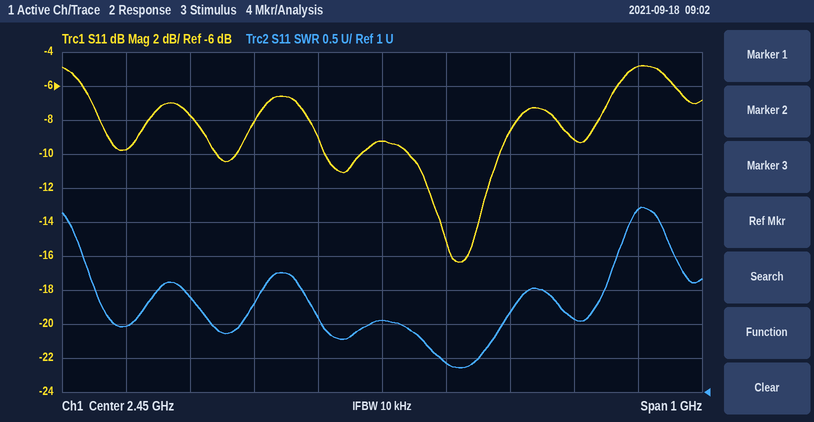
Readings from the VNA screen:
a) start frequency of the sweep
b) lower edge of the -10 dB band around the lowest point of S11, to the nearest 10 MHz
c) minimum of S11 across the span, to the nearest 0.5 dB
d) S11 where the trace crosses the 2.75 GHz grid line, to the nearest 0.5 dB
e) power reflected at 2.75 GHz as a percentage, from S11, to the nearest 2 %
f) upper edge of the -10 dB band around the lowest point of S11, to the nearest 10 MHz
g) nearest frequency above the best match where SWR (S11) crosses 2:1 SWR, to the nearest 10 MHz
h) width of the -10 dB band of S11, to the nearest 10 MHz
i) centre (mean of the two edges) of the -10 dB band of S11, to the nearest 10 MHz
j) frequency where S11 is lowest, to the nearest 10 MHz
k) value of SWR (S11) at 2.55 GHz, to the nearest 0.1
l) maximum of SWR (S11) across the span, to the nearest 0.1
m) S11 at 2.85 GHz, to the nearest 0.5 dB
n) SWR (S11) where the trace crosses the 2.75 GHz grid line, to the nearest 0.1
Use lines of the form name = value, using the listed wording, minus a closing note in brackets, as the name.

start frequency of the sweep = 1.95 GHz
lower edge of the -10 dB band around the lowest point of S11, to the nearest 10 MHz = 2.49 GHz
minimum of S11 across the span, to the nearest 0.5 dB = -16.5 dB
S11 where the trace crosses the 2.75 GHz grid line, to the nearest 0.5 dB = -9.0 dB
power reflected at 2.75 GHz as a percentage, from S11, to the nearest 2 % = 12 %
upper edge of the -10 dB band around the lowest point of S11, to the nearest 10 MHz = 2.63 GHz
nearest frequency above the best match where SWR (S11) crosses 2:1 SWR, to the nearest 10 MHz = 2.64 GHz
width of the -10 dB band of S11, to the nearest 10 MHz = 140 MHz
centre (mean of the two edges) of the -10 dB band of S11, to the nearest 10 MHz = 2.56 GHz
frequency where S11 is lowest, to the nearest 10 MHz = 2.57 GHz
value of SWR (S11) at 2.55 GHz, to the nearest 0.1 = 1.4
maximum of SWR (S11) across the span, to the nearest 0.1 = 3.7
S11 at 2.85 GHz, to the nearest 0.5 dB = -5.0 dB
SWR (S11) where the trace crosses the 2.75 GHz grid line, to the nearest 0.1 = 2.1
